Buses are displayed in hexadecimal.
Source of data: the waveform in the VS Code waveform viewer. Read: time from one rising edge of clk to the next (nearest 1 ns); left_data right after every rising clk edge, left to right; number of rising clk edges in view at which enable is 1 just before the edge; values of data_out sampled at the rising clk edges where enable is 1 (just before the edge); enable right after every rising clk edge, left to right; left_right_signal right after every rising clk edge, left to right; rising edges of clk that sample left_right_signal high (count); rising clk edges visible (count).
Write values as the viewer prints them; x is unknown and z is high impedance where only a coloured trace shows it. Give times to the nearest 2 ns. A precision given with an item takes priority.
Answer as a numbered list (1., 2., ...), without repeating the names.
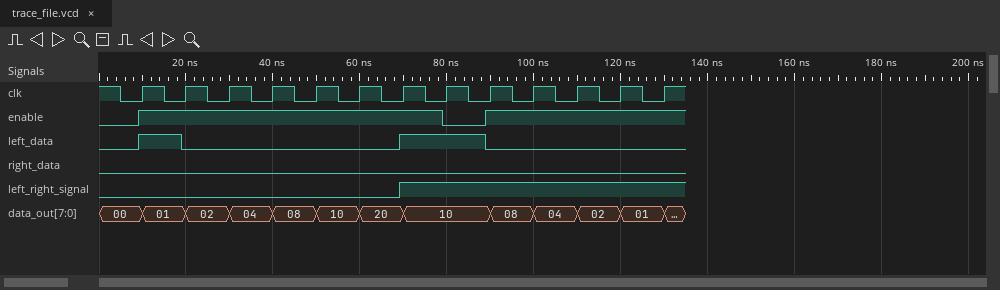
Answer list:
1. 10 ns
2. 1 0 0 0 0 0 1 1 0 0 0 0 0
3. 12
4. 00, 01, 02, 04, 08, 10, 20, 10, 08, 04, 02, 01
5. 1 1 1 1 1 1 1 0 1 1 1 1 1
6. 0 0 0 0 0 0 1 1 1 1 1 1 1
7. 7
8. 13
